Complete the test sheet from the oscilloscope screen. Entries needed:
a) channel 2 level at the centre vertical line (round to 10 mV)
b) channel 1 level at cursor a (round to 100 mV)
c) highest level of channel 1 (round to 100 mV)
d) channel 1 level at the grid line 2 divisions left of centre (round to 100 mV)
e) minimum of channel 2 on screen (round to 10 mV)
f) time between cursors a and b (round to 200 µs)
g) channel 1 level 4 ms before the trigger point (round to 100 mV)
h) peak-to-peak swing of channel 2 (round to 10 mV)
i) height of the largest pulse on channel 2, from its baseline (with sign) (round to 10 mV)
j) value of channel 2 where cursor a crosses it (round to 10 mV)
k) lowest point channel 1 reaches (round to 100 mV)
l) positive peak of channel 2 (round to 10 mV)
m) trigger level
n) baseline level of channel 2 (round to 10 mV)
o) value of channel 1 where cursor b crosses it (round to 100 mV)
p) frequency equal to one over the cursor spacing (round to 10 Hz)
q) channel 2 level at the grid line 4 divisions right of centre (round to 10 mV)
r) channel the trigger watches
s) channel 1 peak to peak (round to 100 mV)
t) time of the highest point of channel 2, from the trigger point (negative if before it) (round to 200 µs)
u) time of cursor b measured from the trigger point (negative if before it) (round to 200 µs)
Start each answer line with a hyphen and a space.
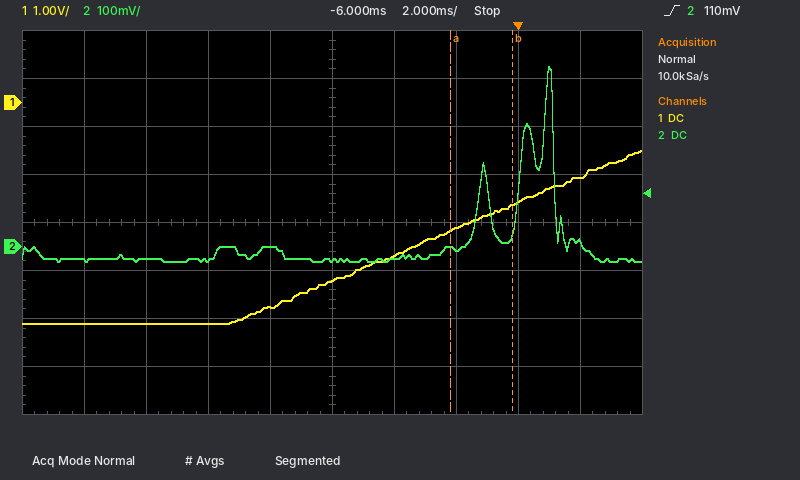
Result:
- -30 mV
- -2.7 V
- -1.0 V
- -4.6 V
- -30 mV
- 2.0 ms
- -3.2 V
- 410 mV
- +400 mV
- 0 mV
- -4.6 V
- 380 mV
- 110 mV
- -20 mV
- -2.1 V
- 500 Hz
- 10 mV
- channel 2
- 3.6 V
- +1.0 ms
- -200 µs
